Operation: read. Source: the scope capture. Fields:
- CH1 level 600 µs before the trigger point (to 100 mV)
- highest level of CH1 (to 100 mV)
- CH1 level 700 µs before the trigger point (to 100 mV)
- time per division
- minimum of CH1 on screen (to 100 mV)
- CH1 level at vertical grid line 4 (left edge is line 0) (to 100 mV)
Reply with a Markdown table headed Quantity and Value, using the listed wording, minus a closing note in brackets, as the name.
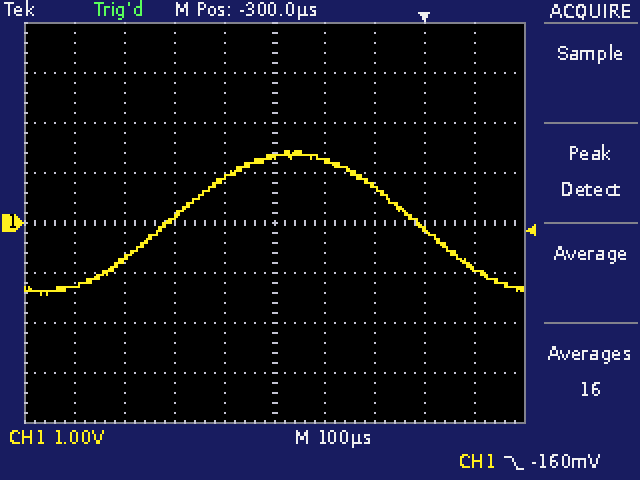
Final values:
| Quantity | Value |
|---|---|
| CH1 level 600 µs before the trigger point | -700 mV |
| highest level of CH1 | 1.4 V |
| CH1 level 700 µs before the trigger point | -1.3 V |
| time per division | 100 µs |
| minimum of CH1 on screen | -1.4 V |
| CH1 level at vertical grid line 4 (left edge is line 0) | 900 mV |
